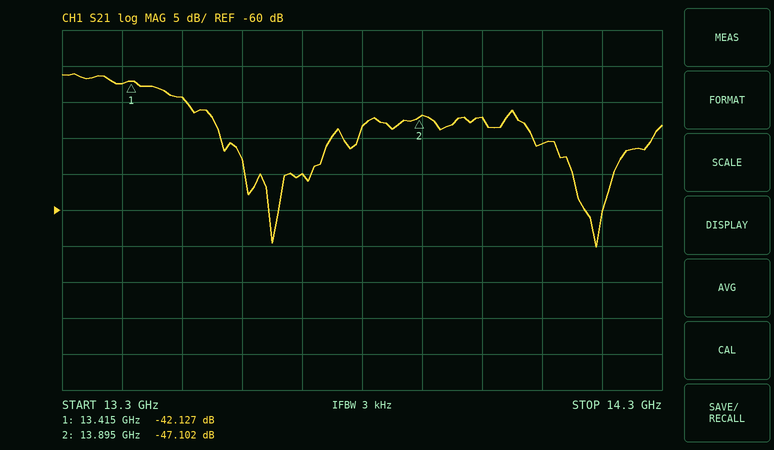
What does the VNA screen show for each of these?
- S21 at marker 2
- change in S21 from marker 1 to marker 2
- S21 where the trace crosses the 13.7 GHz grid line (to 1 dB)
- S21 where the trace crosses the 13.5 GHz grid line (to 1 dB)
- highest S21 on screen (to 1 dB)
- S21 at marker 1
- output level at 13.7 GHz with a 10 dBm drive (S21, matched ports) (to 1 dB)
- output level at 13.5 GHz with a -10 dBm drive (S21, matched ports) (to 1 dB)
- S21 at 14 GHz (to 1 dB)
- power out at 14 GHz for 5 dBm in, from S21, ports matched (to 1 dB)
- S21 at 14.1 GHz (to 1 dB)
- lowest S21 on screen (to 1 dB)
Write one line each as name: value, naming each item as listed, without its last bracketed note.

S21 at marker 2: -47.102 dB
change in S21 from marker 1 to marker 2: -4.975 dB
S21 where the trace crosses the 13.7 GHz grid line: -55 dB
S21 where the trace crosses the 13.5 GHz grid line: -44 dB
highest S21 on screen: -41 dB
S21 at marker 1: -42.127 dB
output level at 13.7 GHz with a 10 dBm drive (S21, matched ports): -45 dBm
output level at 13.5 GHz with a -10 dBm drive (S21, matched ports): -54 dBm
S21 at 14 GHz: -47 dB
power out at 14 GHz for 5 dBm in, from S21, ports matched: -42 dBm
S21 at 14.1 GHz: -51 dB
lowest S21 on screen: -65 dB
